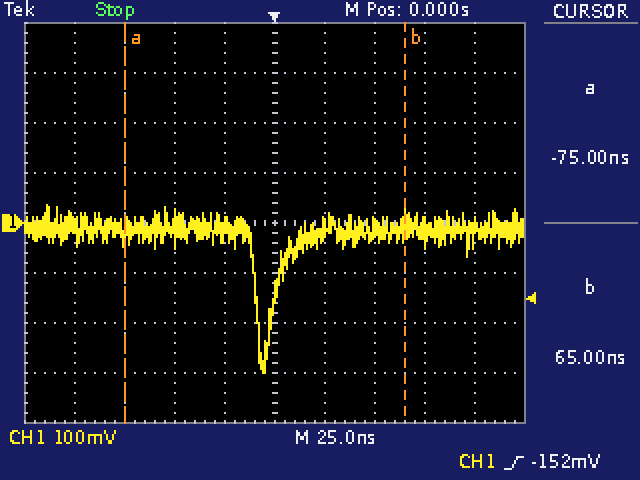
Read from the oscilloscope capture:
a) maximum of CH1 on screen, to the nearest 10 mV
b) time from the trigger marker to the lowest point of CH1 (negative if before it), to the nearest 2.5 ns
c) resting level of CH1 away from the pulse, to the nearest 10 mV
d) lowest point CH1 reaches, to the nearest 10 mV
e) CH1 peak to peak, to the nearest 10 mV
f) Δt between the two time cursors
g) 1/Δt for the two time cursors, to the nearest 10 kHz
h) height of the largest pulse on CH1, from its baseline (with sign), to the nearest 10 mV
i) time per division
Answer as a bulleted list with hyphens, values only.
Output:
- 40 mV
- -5.0 ns
- -10 mV
- -300 mV
- 340 mV
- 140.0 ns
- 7.14 MHz
- -290 mV
- 25 ns
